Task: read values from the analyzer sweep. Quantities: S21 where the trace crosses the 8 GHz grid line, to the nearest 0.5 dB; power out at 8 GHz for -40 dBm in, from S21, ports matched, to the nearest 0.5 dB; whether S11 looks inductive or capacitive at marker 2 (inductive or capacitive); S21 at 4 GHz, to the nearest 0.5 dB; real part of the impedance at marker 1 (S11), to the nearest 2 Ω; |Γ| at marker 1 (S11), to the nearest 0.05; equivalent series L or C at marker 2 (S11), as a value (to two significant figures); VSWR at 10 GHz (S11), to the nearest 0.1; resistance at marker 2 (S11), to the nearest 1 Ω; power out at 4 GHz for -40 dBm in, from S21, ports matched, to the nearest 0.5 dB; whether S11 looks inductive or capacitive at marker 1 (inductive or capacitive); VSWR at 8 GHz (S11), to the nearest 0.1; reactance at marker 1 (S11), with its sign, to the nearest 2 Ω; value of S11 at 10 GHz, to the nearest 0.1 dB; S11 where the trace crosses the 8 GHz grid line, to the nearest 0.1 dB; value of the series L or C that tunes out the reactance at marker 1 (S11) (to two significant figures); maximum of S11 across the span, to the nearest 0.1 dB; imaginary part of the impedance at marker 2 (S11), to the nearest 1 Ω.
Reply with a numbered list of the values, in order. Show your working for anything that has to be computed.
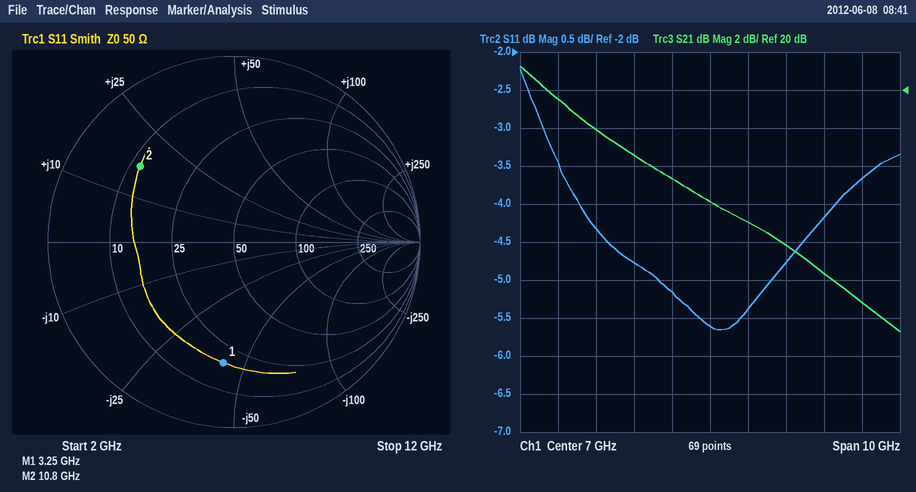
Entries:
1. 13.0 dB
2. -40 dBm + (13.0 dB) = -27.0 dBm
3. inductive
4. 18.0 dB
5. 18 Ω
6. 0.65
7. L = 17 Ω/(2π × 10.8 GHz) ≈ 251 pH, so 250 pH to two significant figures
8. |Γ| = 10^(-4.2/20) = 0.6166; VSWR = (1 + 0.6166)/(1 − 0.6166) ≈ 4.2
9. 12 Ω
10. -40 dBm + (18.0 dB) = -22.0 dBm
11. capacitive
12. |Γ| = 10^(-5.4/20) = 0.5370; VSWR = (1 + 0.5370)/(1 − 0.5370) ≈ 3.3
13. -42 Ω
14. -4.2 dB
15. -5.4 dB
16. L = 42 Ω/(2π × 3.25 GHz) ≈ 2.1 nH
17. -2.2 dB
18. +17 Ω
